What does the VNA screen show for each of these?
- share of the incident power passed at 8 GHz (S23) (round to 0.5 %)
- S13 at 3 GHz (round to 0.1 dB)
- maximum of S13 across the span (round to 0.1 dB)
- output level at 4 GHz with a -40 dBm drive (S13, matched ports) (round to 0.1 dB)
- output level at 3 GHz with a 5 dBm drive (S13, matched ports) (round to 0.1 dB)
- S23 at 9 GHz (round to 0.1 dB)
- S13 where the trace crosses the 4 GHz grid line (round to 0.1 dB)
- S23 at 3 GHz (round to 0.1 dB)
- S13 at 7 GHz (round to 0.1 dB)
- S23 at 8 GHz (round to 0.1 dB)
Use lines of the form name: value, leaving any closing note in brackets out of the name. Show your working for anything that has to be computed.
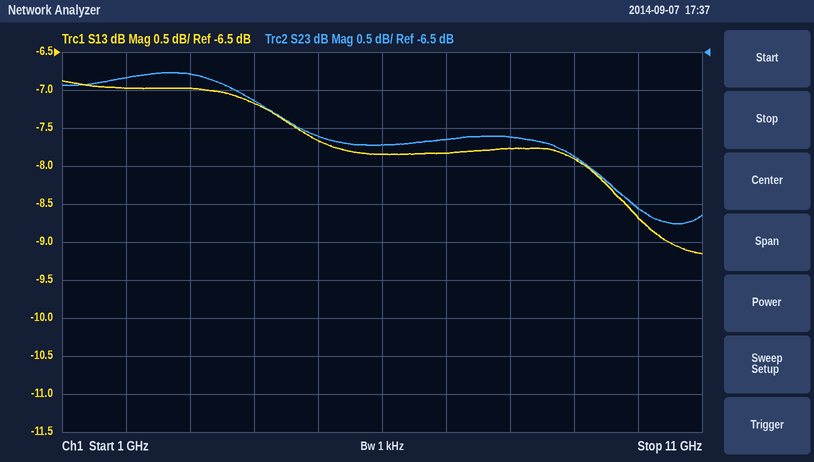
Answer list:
share of the incident power passed at 8 GHz (S23): 10^(-7.6/10) ≈ 17.4 %, so 17.5 % to the nearest 0.5 %
S13 at 3 GHz: -7.0 dB
maximum of S13 across the span: -6.9 dB
output level at 4 GHz with a -40 dBm drive (S13, matched ports): -40 dBm + (-7.2 dB) = -47.2 dBm
output level at 3 GHz with a 5 dBm drive (S13, matched ports): 5 dBm + (-7.0 dB) = -2.0 dBm
S23 at 9 GHz: -7.9 dB
S13 where the trace crosses the 4 GHz grid line: -7.2 dB
S23 at 3 GHz: -6.8 dB
S13 at 7 GHz: -7.8 dB
S23 at 8 GHz: -7.6 dB
